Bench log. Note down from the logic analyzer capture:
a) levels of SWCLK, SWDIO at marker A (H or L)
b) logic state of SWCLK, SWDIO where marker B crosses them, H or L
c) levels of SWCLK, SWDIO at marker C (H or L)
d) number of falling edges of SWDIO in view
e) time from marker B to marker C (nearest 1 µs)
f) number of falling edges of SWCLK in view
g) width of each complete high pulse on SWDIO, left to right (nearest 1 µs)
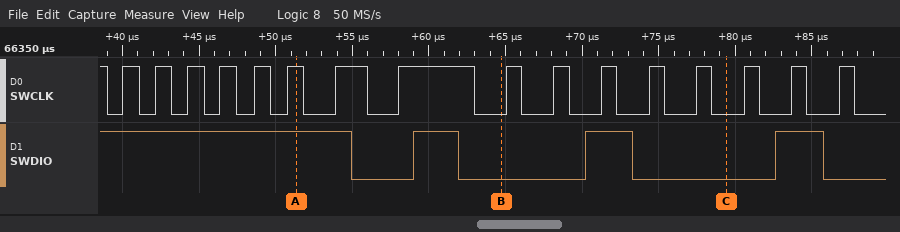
SWCLK=H, SWDIO=H
SWCLK=L, SWDIO=L
SWCLK=L, SWDIO=L
4
15 µs
17
3 µs, 3 µs, 3 µs
